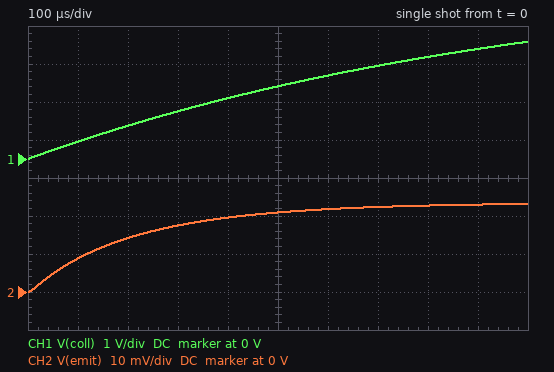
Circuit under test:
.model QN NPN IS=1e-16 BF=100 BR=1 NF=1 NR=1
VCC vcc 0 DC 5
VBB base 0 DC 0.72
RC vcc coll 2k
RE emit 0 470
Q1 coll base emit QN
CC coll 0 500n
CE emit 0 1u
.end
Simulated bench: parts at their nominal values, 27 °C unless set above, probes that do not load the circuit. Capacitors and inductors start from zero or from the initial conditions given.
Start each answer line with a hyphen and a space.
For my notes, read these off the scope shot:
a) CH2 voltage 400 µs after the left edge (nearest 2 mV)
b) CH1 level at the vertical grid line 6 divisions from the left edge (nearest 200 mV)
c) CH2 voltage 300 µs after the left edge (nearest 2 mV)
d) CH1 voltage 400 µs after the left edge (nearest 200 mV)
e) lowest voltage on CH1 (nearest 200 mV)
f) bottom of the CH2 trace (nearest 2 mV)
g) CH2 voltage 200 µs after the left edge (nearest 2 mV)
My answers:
- 20 mV
- 2.2 V
- 18 mV
- 1.6 V
- 0 V
- 0 V
- 14 mV
